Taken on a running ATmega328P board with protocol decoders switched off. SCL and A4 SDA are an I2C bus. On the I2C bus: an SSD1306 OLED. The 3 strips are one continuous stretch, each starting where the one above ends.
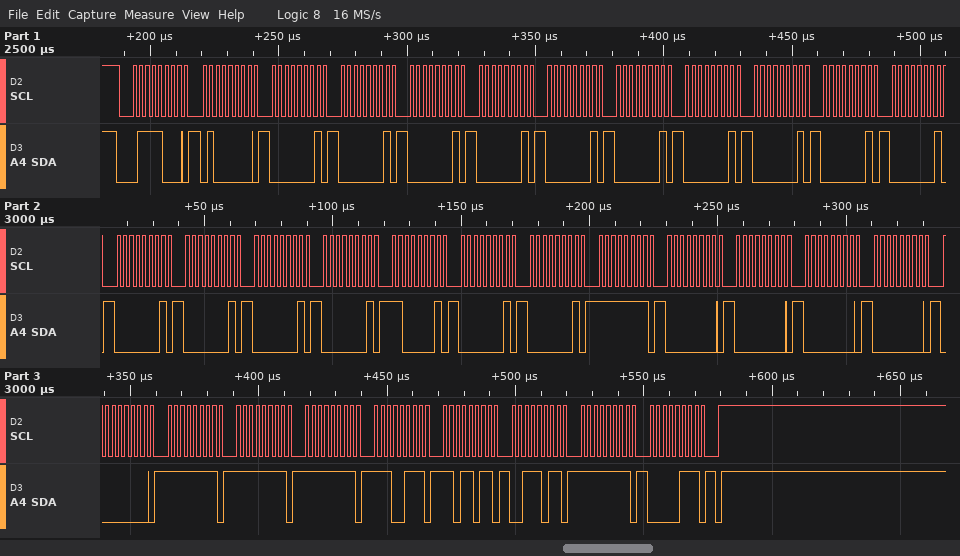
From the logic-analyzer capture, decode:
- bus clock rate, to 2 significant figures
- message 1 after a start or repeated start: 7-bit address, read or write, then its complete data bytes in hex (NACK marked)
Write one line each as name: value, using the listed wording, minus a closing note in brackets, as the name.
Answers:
bus clock rate, to 2 significant figures: 400 kHz
message 1 after a start or repeated start: 7-bit address, read or write, then its complete data bytes in hex: 0x3C write: 40 01 01 01 01 01 01 01 01 01 01 01 01 01 01 C1 01 01 FF 00 00 00 00 00 FF FF FF E7 DB 3B FF 07
